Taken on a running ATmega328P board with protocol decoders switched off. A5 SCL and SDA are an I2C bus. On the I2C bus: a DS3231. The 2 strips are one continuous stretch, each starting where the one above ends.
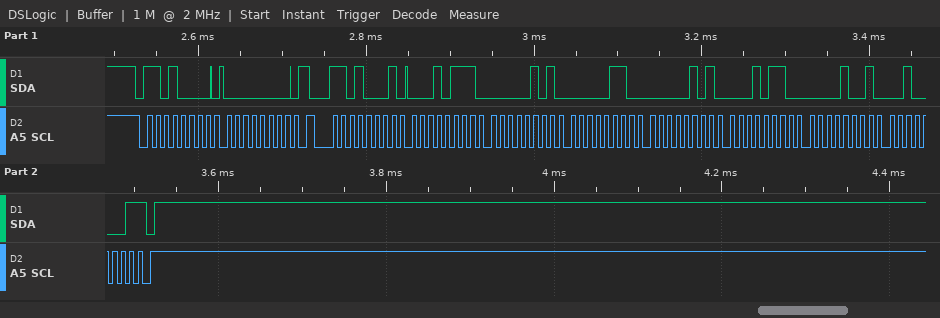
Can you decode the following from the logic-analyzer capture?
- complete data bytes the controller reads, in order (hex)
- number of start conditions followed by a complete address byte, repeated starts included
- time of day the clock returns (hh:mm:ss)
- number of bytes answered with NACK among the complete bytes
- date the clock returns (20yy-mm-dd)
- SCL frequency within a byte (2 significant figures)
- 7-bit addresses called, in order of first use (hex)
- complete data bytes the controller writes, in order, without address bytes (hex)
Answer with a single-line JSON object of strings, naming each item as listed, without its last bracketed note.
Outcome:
{"complete data bytes the controller reads, in order": "17 05 06 05 16 09 21", "number of start conditions followed by a complete address byte, repeated starts included": "2", "time of day the clock returns": "06:05:17", "number of bytes answered with NACK among the complete bytes": "1", "date the clock returns": "2021-09-16", "SCL frequency within a byte": "100 kHz", "7-bit addresses called, in order of first use": "0x68", "complete data bytes the controller writes, in order, without address bytes": "00"}
